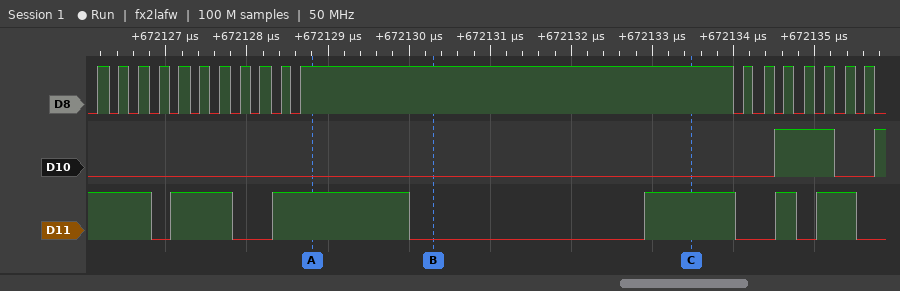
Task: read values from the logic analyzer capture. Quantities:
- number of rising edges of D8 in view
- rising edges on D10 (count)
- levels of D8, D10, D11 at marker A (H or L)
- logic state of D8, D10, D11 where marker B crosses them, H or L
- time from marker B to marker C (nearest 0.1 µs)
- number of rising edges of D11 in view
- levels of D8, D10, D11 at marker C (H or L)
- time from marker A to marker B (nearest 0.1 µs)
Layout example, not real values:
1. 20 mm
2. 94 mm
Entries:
1. 18
2. 2
3. D8=H, D10=L, D11=H
4. D8=H, D10=L, D11=L
5. 3.2 µs
6. 5
7. D8=H, D10=L, D11=H
8. 1.5 µs
